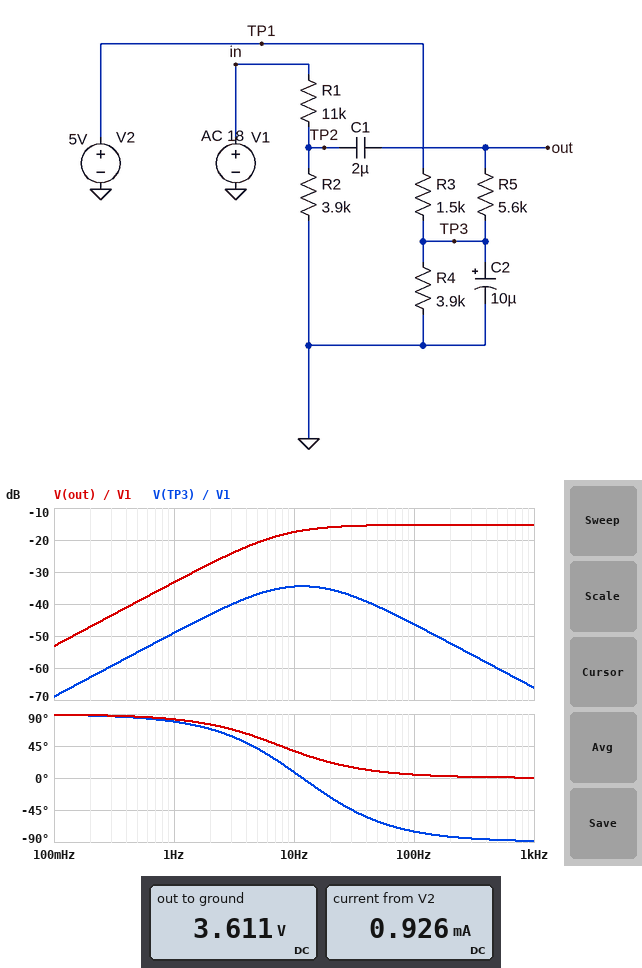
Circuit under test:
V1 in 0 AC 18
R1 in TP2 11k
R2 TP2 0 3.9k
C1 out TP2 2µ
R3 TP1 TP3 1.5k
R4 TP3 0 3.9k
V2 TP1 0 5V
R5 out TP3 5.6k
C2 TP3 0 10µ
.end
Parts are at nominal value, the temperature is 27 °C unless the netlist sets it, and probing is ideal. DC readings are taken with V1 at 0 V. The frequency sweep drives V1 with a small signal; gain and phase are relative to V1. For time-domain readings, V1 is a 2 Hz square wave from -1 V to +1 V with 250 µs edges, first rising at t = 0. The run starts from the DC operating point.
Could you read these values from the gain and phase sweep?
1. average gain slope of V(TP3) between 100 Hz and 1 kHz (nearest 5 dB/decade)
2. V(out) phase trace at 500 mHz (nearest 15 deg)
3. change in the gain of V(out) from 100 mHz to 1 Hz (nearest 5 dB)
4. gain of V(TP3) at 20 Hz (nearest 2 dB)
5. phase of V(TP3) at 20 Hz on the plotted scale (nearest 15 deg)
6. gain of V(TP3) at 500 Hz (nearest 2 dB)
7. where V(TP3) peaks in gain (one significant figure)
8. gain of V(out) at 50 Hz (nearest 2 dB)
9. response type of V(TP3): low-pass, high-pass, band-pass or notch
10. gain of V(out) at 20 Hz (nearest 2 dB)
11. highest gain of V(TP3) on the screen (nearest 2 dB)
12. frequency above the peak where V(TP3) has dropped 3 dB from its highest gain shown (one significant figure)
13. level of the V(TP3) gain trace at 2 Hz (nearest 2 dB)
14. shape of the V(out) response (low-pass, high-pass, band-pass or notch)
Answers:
-20 dB/decade
90 deg
20 dB
-36 dB
-30 deg
-60 dB
10 Hz
-16 dB
band-pass
-16 dB
-34 dB
30 Hz
-44 dB
high-pass
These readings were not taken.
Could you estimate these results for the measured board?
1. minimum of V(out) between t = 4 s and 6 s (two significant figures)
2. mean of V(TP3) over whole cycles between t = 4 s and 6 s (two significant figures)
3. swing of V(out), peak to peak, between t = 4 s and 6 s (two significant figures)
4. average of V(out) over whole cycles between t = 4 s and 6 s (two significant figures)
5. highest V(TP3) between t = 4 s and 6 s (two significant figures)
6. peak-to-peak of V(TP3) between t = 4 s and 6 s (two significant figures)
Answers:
3.3 V
3.6 V
690 mV
3.6 V
3.6 V
58 mV
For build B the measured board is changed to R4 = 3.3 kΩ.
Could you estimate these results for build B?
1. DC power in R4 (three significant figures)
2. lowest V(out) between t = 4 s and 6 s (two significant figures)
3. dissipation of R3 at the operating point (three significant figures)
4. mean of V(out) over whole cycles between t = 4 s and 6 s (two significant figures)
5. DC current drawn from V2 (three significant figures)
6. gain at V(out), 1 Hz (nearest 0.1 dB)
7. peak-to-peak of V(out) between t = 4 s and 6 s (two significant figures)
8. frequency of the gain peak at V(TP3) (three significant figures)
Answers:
3.58 mW
3.1 V
1.63 mW
3.4 V
1.04 mA
-33.3 dB
690 mV
12.0 Hz
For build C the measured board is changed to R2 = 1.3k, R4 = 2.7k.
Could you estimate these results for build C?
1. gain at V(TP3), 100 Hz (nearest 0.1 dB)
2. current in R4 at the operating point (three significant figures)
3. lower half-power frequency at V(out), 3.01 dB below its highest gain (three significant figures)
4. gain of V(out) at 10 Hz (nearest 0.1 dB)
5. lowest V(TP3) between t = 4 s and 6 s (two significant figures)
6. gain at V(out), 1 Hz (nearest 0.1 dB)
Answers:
-52.3 dB
1.19 mA
10.9 Hz
-24.5 dB
3.2 V
-41.2 dB
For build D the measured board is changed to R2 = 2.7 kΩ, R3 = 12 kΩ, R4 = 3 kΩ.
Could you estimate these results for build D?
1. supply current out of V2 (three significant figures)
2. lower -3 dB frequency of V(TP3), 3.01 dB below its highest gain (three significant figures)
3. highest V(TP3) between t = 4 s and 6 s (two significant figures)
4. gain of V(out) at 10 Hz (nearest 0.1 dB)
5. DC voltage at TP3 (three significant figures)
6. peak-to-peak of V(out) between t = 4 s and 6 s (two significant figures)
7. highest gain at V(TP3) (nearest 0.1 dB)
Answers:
333 µA
3.09 Hz
1.0 V
-19.8 dB
1.00 V
560 mV
-33.4 dB
